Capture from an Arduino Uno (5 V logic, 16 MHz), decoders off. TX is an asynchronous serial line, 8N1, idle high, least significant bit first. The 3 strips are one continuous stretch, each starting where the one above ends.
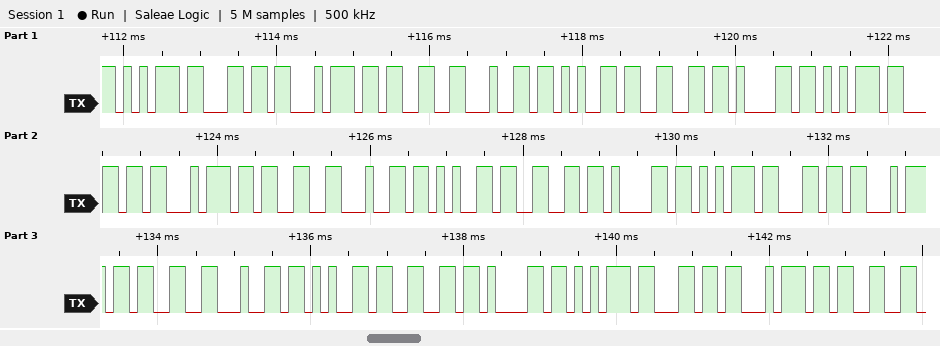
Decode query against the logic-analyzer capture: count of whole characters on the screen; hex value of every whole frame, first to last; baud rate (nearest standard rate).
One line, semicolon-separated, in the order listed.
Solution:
28; 75 6C 74 33 64 65 66 61 75 6C 74 33 64 65 66 61 75 6C 74 33 64 65 66 61 75 6C 74 33; 9600 baud
